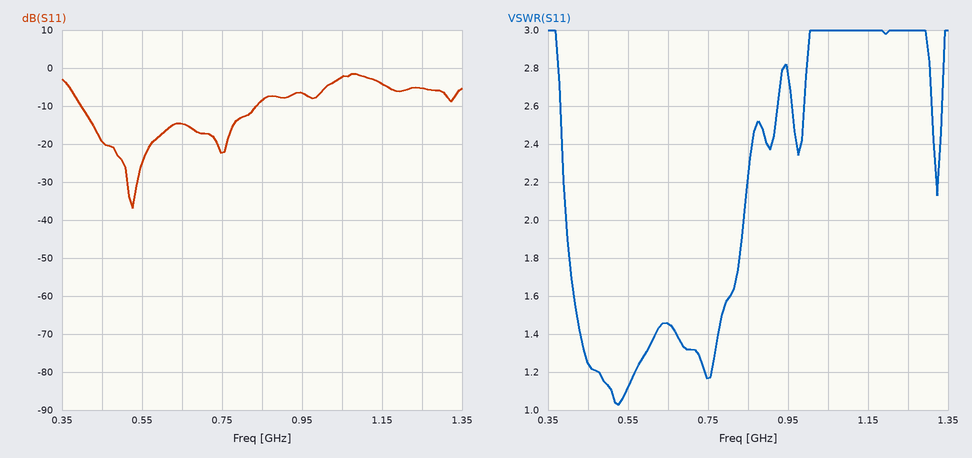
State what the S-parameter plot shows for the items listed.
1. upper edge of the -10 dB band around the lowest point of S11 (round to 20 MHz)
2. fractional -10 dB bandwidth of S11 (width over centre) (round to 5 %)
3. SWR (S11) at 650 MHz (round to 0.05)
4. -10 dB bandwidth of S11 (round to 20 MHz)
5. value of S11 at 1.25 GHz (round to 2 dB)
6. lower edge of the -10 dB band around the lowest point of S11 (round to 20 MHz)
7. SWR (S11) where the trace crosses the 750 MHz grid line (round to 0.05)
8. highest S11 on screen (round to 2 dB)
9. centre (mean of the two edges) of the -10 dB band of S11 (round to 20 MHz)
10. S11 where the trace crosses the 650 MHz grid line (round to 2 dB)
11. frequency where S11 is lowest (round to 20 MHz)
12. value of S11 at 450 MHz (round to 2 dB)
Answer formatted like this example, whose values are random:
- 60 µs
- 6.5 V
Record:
- 840 MHz
- 70 %
- 1.45
- 440 MHz
- -6 dB
- 400 MHz
- 1.15
- -2 dB
- 620 MHz
- -14 dB
- 520 MHz
- -20 dB
